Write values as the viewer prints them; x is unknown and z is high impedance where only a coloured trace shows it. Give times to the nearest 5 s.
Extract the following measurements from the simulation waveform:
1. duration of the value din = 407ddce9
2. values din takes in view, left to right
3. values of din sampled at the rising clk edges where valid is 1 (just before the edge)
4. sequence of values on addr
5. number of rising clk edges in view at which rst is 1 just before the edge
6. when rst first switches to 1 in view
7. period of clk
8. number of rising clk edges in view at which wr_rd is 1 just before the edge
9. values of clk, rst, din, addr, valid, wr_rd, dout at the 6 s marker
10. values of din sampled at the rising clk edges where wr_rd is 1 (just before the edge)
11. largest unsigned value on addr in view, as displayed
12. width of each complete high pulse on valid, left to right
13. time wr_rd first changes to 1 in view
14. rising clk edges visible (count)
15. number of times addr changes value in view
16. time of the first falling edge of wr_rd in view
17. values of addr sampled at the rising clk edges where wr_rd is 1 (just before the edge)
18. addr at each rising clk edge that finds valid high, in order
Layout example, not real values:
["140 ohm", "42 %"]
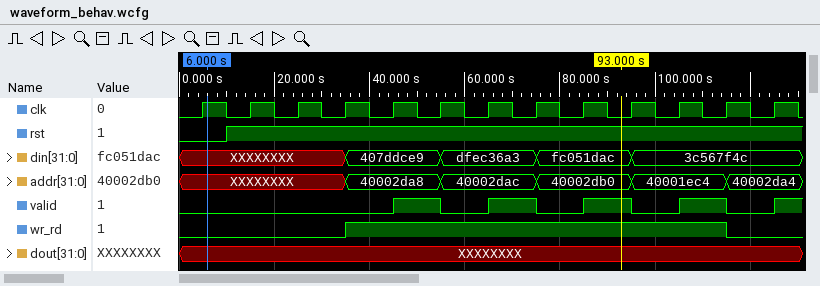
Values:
["20 s", "XXXXXXXX, 407ddce9, dfec36a3, fc051dac, 3c567f4c", "407ddce9, dfec36a3, fc051dac, 3c567f4c", "XXXXXXXX, 40002da8, 40002dac, 40002db0, 40001ec4, 40002da4", "12", "10 s", "10 s", "8", "clk=1, rst=0, din=XXXXXXXX, addr=XXXXXXXX, valid=0, wr_rd=0, dout=XXXXXXXX", "407ddce9, 407ddce9, dfec36a3, dfec36a3, fc051dac, fc051dac, 3c567f4c, 3c567f4c", "40002db0", "10 s, 10 s, 10 s, 10 s", "35 s", "13", "5", "115 s", "40002da8, 40002da8, 40002dac, 40002dac, 40002db0, 40002db0, 40001ec4, 40001ec4", "40002da8, 40002dac, 40002db0, 40001ec4"]
